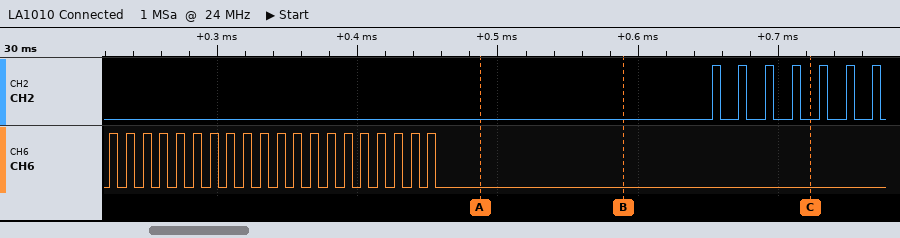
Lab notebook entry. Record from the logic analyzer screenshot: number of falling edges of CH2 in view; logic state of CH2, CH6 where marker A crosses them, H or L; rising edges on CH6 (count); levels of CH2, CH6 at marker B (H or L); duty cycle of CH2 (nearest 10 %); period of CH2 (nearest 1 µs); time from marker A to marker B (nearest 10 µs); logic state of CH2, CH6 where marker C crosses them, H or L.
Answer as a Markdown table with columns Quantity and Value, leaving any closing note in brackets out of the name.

| Quantity | Value |
|---|---|
| number of falling edges of CH2 in view | 7 |
| logic state of CH2, CH6 where marker A crosses them, H or L | CH2=L, CH6=L |
| rising edges on CH6 | 20 |
| levels of CH2, CH6 at marker B | CH2=L, CH6=L |
| duty cycle of CH2 | 30 % |
| period of CH2 | 19 µs |
| time from marker A to marker B | 100 µs |
| logic state of CH2, CH6 where marker C crosses them, H or L | CH2=L, CH6=L |
